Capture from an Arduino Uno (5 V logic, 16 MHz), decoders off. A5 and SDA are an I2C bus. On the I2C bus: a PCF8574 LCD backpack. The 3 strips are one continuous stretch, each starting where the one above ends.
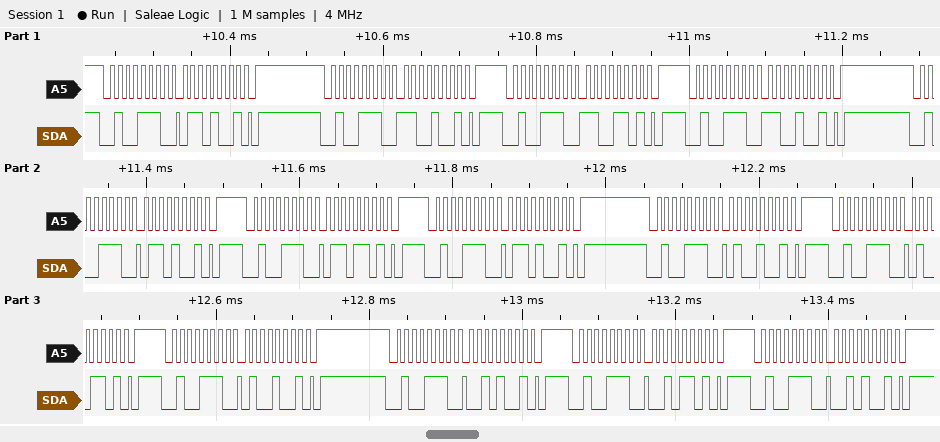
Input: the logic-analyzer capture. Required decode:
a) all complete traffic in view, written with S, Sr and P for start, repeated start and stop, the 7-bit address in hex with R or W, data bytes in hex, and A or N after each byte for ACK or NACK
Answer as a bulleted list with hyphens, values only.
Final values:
- S 27W A 69 A P S 27W A C9 A P S 27W A CD A P S 27W A C9 A P S 27W A 69 A P S 27W A 6D A P S 27W A 69 A P S 27W A 49 A P S 27W A 4D A P S 27W A 49 A P S 27W A 29 A P S 27W A 2D A P S 27W A 29 A P
